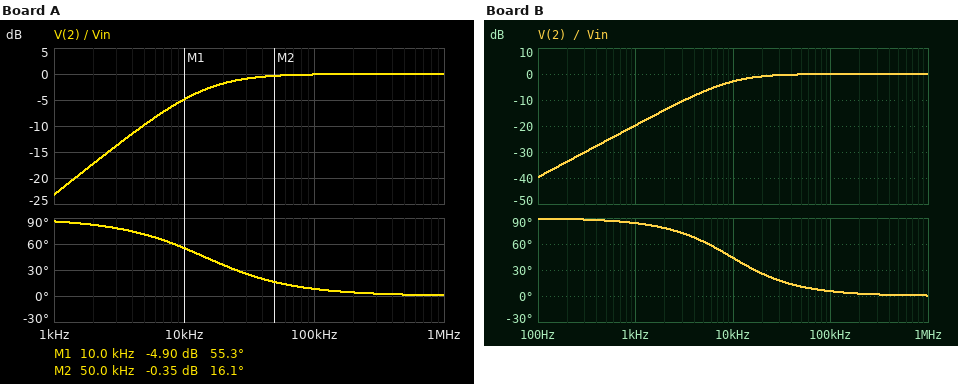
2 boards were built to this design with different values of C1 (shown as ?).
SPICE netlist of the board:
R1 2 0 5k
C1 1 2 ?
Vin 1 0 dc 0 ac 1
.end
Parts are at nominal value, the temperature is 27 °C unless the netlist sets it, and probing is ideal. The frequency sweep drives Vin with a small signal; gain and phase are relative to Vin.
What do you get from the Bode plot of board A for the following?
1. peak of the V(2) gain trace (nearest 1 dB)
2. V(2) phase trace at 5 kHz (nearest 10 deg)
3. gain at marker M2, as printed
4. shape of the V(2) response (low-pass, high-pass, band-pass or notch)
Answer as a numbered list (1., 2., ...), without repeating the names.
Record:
1. 0 dB
2. 70 deg
3. -0.35 dB
4. high-pass
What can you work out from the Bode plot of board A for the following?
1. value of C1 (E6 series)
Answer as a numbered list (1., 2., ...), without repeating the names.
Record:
1. 2.2 nF
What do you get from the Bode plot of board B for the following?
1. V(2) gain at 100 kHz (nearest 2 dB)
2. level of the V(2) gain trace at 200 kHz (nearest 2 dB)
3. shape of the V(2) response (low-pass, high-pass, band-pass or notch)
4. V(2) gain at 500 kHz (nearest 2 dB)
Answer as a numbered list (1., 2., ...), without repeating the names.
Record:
1. 0 dB
2. 0 dB
3. high-pass
4. 0 dB
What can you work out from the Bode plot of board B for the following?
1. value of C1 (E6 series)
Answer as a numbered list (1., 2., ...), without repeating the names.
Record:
1. 3.3 nF
